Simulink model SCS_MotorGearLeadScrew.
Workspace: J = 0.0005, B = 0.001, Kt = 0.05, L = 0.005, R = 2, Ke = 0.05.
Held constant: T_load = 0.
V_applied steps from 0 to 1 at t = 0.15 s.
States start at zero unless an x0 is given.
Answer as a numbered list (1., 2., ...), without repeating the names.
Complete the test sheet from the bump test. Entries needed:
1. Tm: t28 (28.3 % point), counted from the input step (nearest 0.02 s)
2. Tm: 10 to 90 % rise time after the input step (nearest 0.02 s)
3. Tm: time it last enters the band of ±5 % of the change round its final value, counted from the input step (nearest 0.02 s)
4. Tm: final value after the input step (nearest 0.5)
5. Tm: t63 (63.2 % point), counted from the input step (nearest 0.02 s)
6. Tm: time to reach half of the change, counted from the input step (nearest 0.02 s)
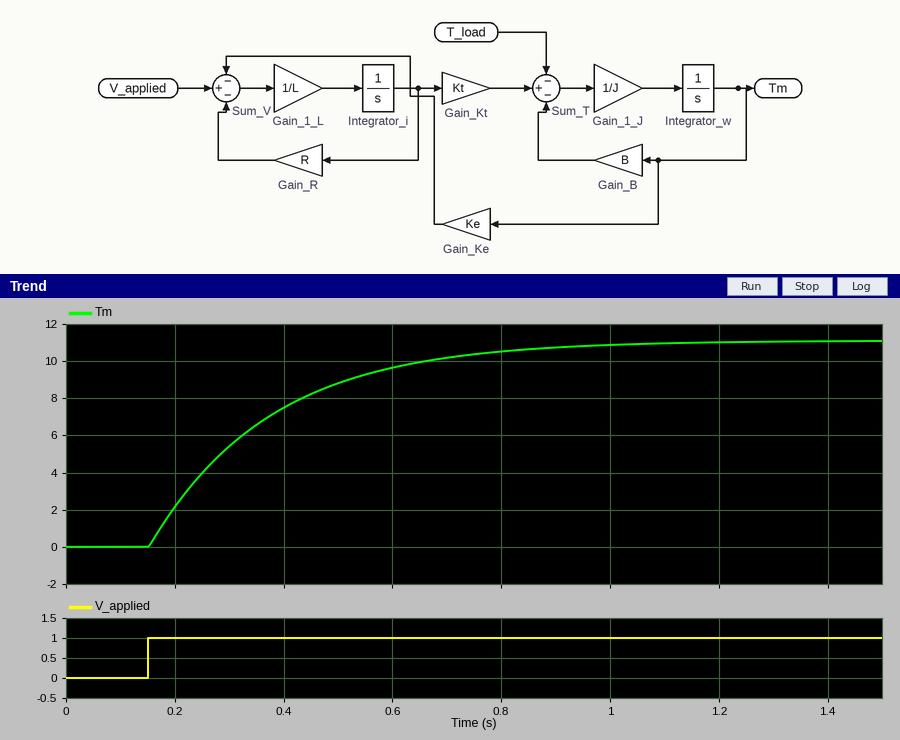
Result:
1. 0.08 s
2. 0.48 s
3. 0.66 s
4. 11.0
5. 0.22 s
6. 0.16 s
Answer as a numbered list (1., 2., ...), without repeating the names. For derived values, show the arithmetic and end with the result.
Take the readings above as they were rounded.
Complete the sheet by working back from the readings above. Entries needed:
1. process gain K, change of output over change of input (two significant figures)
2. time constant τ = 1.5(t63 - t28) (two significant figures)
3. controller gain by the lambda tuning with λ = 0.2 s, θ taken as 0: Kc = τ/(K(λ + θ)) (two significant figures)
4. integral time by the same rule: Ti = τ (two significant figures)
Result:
1. (11 - 0) / 1 = 11
2. 1.5 × (0.22 - 0.08) = 0.21 s
3. 0.21 / (11 × (0.2 + 0)) = 0.095
4. 0.21 s
